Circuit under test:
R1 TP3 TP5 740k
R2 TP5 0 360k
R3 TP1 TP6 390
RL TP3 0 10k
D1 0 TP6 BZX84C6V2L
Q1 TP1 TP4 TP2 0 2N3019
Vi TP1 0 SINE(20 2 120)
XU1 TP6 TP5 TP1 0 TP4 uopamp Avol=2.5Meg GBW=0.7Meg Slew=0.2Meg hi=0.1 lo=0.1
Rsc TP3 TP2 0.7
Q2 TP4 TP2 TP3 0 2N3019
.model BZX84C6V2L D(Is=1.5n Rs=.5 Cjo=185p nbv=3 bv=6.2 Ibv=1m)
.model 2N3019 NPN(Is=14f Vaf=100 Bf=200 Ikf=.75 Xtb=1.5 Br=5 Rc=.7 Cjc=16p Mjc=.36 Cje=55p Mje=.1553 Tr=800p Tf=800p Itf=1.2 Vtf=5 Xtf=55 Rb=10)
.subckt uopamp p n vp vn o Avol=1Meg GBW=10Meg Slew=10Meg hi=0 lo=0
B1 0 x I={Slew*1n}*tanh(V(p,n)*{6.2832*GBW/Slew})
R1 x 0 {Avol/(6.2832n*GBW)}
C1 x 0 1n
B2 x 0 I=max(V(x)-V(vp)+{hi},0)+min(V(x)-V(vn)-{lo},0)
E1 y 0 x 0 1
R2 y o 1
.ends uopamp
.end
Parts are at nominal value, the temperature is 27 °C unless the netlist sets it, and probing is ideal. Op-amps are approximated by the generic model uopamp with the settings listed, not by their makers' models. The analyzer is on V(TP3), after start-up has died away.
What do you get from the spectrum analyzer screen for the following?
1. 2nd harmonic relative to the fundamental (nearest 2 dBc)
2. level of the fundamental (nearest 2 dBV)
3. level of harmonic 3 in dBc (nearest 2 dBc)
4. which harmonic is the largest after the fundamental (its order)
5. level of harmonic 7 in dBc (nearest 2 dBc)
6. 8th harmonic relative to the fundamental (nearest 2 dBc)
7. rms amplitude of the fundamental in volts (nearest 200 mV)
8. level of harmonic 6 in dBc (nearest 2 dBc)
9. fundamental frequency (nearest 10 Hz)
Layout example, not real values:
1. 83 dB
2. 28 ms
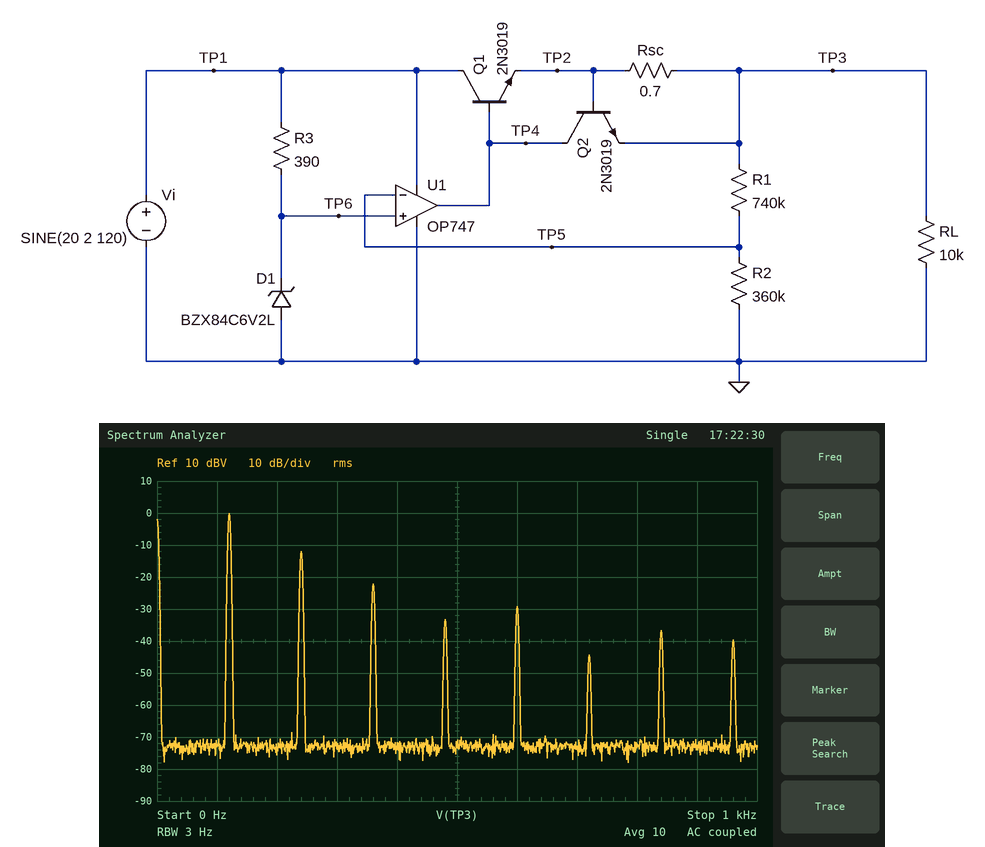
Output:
1. -12 dBc
2. 0 dBV
3. -22 dBc
4. 2
5. -36 dBc
6. -40 dBc
7. 1.0 V
8. -44 dBc
9. 120 Hz
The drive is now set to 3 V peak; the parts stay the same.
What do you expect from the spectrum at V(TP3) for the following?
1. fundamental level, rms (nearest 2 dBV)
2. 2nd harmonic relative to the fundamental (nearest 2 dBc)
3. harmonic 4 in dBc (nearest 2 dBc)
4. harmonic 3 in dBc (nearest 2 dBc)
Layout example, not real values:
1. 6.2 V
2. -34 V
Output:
1. 2 dBV
2. -10 dBc
3. -26 dBc
4. -24 dBc
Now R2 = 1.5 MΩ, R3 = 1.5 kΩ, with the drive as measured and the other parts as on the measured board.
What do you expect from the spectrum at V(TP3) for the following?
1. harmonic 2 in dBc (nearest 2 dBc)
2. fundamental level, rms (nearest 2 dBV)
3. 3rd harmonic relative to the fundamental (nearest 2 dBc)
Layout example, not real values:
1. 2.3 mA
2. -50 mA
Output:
1. -30 dBc
2. -38 dBV
3. -56 dBc
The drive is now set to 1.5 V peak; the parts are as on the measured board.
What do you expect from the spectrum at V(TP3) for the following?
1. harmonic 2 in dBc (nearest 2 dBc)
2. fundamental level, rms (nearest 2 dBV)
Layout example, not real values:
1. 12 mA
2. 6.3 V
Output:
1. -14 dBc
2. -2 dBV
